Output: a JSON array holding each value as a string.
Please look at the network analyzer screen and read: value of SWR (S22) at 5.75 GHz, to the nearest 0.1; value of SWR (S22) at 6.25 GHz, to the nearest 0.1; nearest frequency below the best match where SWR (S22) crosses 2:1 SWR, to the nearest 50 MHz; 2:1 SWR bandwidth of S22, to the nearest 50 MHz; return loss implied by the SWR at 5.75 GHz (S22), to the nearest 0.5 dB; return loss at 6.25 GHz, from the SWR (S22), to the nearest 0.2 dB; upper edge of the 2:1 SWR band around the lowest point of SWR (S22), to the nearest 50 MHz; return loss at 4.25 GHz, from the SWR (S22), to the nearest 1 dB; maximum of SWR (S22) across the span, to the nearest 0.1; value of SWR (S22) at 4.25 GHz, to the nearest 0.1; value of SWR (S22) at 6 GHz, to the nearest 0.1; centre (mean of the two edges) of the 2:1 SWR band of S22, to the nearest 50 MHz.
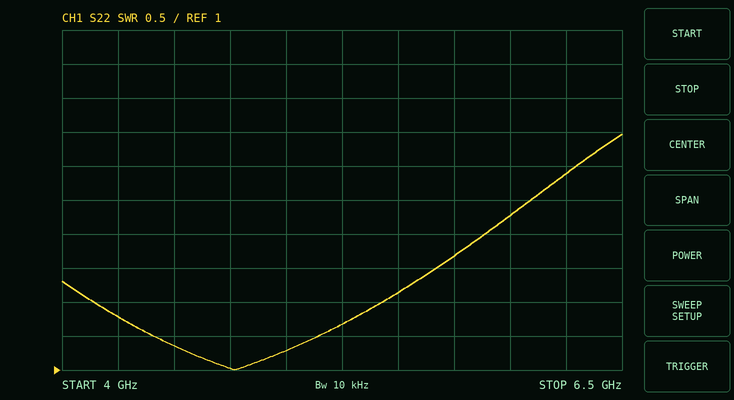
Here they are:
["2.7", "3.9", "4.15 GHz", "1.30 GHz", "7.0 dB", "4.6 dB", "5.45 GHz", "11 dB", "4.5", "1.8", "3.3", "4.80 GHz"]
